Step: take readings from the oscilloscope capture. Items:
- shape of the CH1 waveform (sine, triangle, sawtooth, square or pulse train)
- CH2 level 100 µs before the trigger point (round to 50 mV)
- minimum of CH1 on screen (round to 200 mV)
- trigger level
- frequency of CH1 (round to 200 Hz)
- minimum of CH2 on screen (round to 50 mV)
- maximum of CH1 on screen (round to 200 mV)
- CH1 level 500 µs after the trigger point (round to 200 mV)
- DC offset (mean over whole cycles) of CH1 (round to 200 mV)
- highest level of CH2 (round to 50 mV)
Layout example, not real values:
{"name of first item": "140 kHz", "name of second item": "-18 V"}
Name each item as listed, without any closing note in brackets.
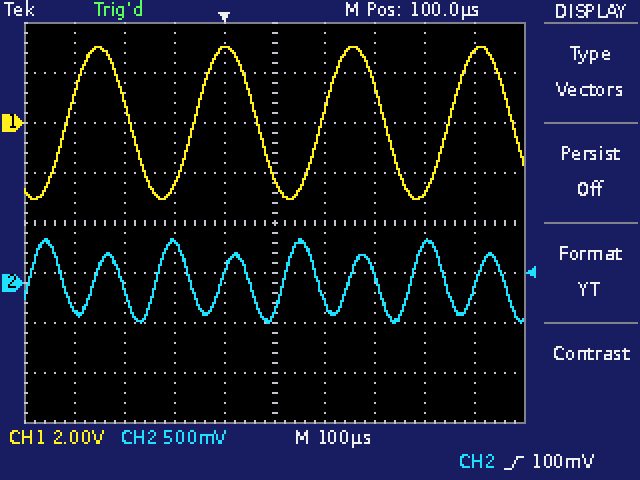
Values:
{"shape of the CH1 waveform": "sine", "CH2 level 100 µs before the trigger point": "400 mV", "minimum of CH1 on screen": "-3.0 V", "trigger level": "100 mV", "frequency of CH1": "4.0 kHz", "minimum of CH2 on screen": "-400 mV", "maximum of CH1 on screen": "3.0 V", "CH1 level 500 µs after the trigger point": "2.8 V", "DC offset (mean over whole cycles) of CH1": "0.0 V", "highest level of CH2": "450 mV"}
